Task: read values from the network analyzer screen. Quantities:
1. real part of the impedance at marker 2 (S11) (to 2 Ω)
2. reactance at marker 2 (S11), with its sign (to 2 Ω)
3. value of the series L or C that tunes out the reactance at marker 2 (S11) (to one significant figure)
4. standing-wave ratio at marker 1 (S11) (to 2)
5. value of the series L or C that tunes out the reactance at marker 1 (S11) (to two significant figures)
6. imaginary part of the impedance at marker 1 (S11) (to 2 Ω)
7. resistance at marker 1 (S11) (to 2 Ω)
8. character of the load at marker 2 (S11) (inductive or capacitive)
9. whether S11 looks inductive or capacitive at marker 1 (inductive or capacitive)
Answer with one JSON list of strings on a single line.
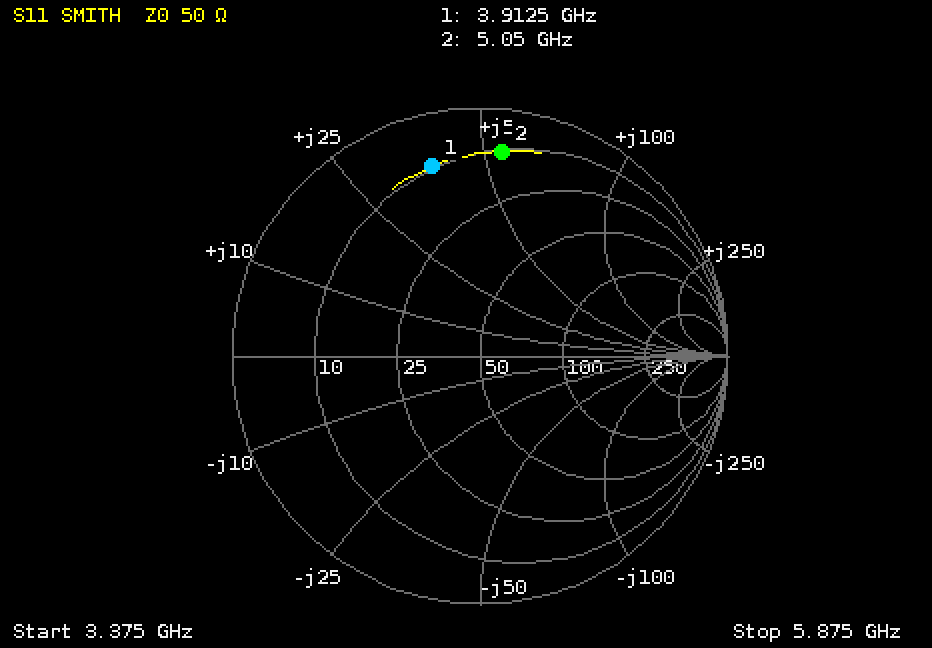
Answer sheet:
["10 Ω", "+54 Ω", "600 fF", "8", "1.1 pF", "+38 Ω", "10 Ω", "inductive", "inductive"]
